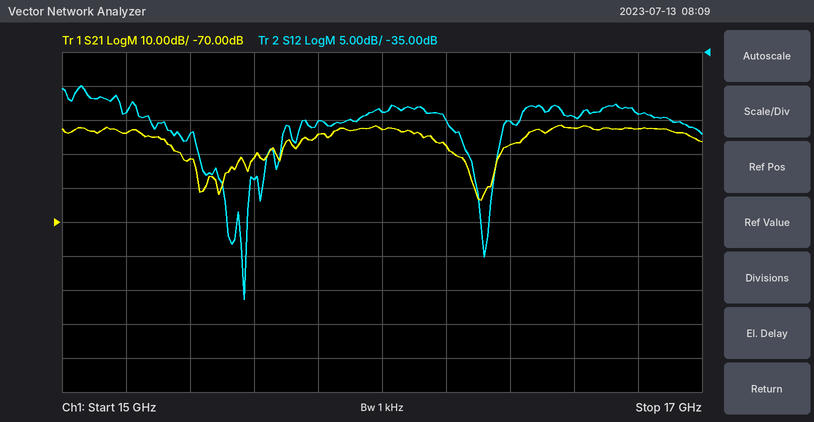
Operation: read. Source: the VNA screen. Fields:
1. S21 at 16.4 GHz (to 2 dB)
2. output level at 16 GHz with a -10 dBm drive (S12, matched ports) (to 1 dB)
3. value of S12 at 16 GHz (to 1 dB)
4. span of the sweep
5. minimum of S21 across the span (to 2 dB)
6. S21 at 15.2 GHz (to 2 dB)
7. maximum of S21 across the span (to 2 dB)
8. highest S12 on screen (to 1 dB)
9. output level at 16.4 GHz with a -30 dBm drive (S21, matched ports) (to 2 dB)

-48 dB
-54 dBm
-44 dB
2 GHz
-64 dB
-44 dB
-42 dB
-40 dB
-78 dBm
